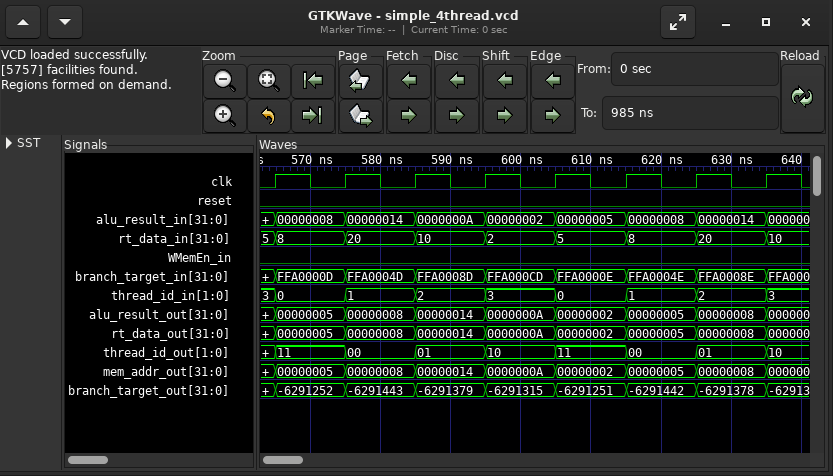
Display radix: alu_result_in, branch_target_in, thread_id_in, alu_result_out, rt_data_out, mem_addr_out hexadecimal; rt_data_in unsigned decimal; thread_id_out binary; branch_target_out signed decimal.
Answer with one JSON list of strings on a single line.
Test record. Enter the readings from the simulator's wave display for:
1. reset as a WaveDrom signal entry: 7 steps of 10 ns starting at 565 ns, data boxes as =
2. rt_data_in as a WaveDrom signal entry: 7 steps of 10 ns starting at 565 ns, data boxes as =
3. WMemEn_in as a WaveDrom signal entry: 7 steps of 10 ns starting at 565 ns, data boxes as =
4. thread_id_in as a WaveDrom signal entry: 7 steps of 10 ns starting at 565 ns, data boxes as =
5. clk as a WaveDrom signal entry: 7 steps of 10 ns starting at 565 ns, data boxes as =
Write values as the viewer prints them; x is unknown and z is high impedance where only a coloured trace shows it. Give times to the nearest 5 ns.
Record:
["{name: 'reset', wave: '0......'}", "{name: 'rt_data_in', wave: '=======', data: '8 20 10 2 5 8 20'}", "{name: 'WMemEn_in', wave: '0......'}", "{name: 'thread_id_in', wave: '=======', data: '0 1 2 3 0 1 2'}", "{name: 'clk', wave: 'p......'}"]
